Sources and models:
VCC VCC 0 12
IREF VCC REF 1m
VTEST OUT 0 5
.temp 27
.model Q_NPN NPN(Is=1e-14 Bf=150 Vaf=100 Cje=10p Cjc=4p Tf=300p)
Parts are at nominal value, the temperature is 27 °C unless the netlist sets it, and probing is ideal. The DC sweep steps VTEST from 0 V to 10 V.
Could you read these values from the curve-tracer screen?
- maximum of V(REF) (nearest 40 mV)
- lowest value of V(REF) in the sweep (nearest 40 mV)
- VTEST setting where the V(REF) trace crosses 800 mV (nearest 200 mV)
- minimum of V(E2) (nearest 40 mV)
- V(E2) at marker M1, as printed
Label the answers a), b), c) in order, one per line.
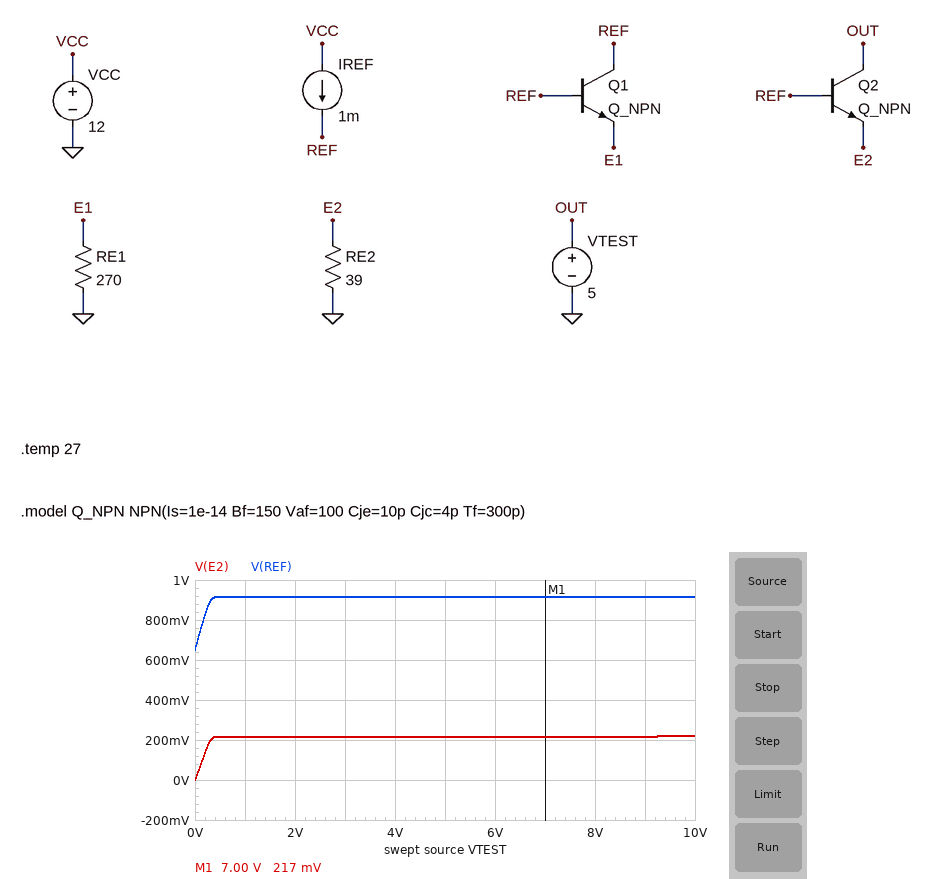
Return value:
a) 920 mV
b) 640 mV
c) 200 mV
d) 0 V
e) 217 mV
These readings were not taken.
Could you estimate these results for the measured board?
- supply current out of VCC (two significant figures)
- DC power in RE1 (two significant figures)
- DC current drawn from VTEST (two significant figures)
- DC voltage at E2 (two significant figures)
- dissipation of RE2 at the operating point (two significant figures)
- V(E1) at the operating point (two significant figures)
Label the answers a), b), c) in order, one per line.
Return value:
a) 1.0 mA
b) 250 µW
c) 5.5 mA
d) 220 mV
e) 1.2 mW
f) 260 mV
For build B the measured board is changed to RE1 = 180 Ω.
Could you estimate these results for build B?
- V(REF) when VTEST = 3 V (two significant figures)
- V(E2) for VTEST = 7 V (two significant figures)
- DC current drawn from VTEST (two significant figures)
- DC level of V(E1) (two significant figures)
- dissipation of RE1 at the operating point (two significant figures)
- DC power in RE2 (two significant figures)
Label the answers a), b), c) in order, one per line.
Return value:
a) 830 mV
b) 140 mV
c) 3.6 mA
d) 180 mV
e) 170 µW
f) 520 µW
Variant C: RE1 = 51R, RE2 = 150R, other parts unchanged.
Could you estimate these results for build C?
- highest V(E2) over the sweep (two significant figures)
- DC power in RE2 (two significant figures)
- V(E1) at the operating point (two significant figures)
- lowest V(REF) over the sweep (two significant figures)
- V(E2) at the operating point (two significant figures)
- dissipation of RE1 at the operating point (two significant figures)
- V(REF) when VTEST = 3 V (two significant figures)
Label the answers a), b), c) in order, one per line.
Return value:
a) 72 mV
b) 34 µW
c) 51 mV
d) 640 mV
e) 71 mV
f) 51 µW
g) 710 mV
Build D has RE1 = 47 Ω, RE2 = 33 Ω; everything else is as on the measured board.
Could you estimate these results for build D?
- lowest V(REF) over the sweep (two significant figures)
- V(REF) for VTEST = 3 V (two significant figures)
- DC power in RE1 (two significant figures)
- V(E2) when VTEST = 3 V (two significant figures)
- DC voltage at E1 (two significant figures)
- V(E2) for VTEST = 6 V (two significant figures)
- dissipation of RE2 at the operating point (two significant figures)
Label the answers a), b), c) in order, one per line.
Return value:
a) 640 mV
b) 700 mV
c) 46 µW
d) 41 mV
e) 47 mV
f) 42 mV
g) 52 µW
